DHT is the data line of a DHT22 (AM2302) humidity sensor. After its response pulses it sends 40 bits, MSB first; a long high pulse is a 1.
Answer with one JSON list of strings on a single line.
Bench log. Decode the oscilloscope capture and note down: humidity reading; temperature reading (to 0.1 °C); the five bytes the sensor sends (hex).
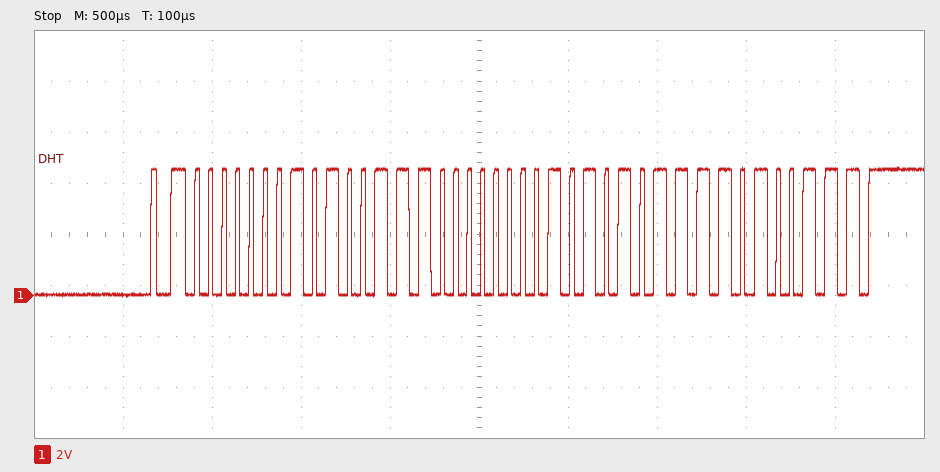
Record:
["33.4 %", "34.3 °C", "01 4E 01 57 A7"]
